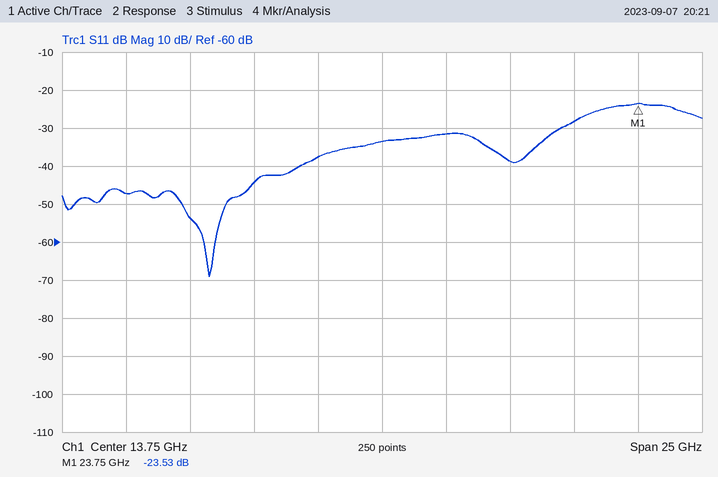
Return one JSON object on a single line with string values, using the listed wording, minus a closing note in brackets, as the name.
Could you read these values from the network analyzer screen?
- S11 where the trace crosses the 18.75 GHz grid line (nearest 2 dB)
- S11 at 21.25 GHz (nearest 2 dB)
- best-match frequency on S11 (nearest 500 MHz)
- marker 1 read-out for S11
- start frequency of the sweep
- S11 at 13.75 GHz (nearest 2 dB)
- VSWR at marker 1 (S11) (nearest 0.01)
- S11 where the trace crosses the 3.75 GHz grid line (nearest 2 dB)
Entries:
{"S11 where the trace crosses the 18.75 GHz grid line": "-38 dB", "S11 at 21.25 GHz": "-28 dB", "best-match frequency on S11": "7.0 GHz", "marker 1 read-out for S11": "-23.53 dB", "start frequency of the sweep": "1.25 GHz", "S11 at 13.75 GHz": "-34 dB", "VSWR at marker 1 (S11)": "1.14", "S11 where the trace crosses the 3.75 GHz grid line": "-48 dB"}
